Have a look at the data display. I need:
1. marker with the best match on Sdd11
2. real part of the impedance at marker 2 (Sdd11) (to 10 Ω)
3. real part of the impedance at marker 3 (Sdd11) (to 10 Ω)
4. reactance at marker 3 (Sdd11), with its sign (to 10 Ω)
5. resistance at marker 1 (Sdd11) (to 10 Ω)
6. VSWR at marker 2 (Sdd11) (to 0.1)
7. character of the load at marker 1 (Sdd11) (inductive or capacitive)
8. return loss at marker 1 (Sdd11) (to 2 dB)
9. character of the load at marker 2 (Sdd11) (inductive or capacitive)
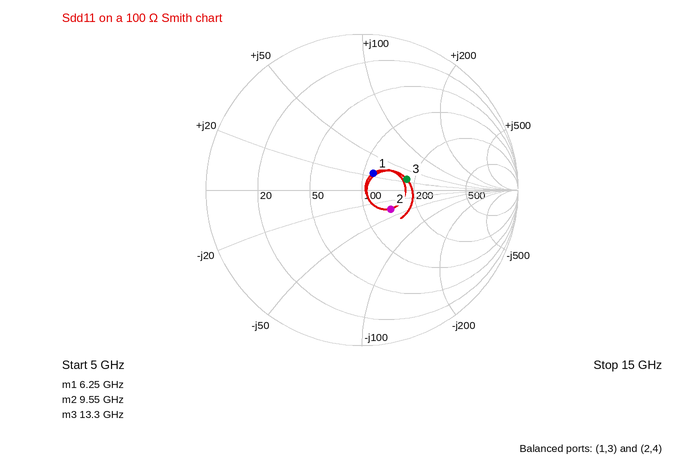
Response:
marker 1
140 Ω
180 Ω
+30 Ω
110 Ω
1.6
inductive
18 dB
capacitive
